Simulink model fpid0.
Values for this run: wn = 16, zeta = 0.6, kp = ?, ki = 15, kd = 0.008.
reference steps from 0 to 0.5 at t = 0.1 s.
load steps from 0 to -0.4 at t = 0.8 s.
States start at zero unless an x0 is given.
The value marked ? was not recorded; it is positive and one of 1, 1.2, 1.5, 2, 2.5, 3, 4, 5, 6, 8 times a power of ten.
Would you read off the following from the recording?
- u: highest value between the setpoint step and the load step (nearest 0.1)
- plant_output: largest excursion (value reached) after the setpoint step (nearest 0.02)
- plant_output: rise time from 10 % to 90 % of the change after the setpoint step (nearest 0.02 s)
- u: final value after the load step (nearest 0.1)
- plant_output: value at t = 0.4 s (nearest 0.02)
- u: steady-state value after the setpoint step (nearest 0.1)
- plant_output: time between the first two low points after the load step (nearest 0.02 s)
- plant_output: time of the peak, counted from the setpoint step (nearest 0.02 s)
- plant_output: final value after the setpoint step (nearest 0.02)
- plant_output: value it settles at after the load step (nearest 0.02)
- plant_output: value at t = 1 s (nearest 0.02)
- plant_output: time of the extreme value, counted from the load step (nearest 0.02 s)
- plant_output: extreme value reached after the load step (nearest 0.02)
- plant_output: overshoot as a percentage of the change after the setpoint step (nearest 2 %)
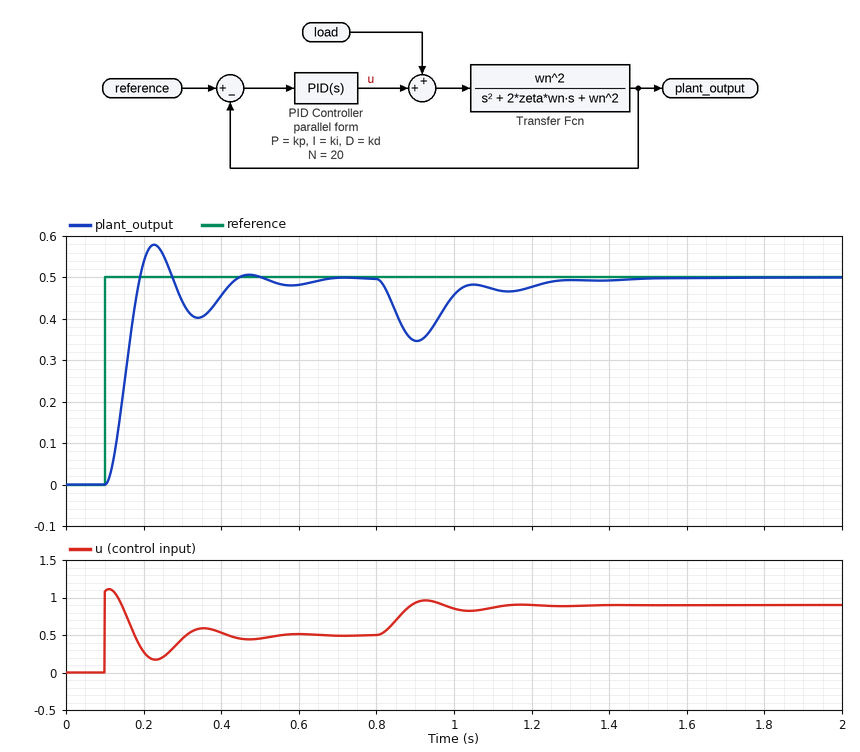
1.1
0.58
0.06 s
0.9
0.46
0.5
0.24 s
0.12 s
0.50
0.50
0.46
0.10 s
0.34
16 %
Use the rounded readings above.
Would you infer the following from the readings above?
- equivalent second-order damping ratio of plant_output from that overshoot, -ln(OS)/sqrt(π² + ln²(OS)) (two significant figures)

0.50
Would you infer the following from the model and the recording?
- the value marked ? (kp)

2
